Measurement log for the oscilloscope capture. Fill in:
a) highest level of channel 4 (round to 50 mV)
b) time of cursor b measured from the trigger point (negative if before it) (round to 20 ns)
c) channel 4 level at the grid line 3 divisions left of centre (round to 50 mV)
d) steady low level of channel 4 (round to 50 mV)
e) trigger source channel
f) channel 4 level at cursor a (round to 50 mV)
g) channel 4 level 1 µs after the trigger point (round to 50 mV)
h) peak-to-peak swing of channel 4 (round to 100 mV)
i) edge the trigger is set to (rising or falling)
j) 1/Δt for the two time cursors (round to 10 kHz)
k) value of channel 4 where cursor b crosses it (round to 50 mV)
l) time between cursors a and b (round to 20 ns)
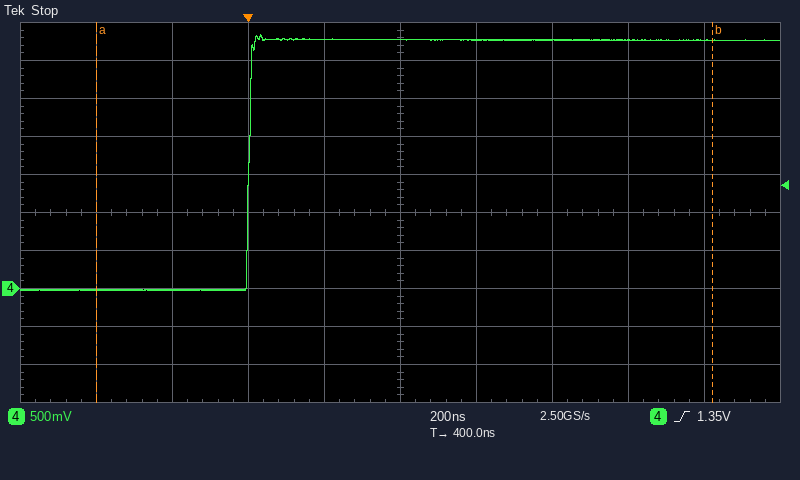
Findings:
3.35 V
+1.22 µs
0 mV
0 mV
channel 4
0 mV
3.25 V
3.40 V
rising
620 kHz
3.25 V
1.62 µs
